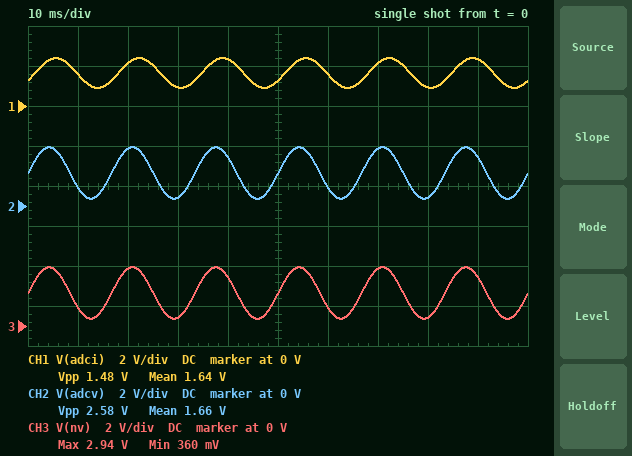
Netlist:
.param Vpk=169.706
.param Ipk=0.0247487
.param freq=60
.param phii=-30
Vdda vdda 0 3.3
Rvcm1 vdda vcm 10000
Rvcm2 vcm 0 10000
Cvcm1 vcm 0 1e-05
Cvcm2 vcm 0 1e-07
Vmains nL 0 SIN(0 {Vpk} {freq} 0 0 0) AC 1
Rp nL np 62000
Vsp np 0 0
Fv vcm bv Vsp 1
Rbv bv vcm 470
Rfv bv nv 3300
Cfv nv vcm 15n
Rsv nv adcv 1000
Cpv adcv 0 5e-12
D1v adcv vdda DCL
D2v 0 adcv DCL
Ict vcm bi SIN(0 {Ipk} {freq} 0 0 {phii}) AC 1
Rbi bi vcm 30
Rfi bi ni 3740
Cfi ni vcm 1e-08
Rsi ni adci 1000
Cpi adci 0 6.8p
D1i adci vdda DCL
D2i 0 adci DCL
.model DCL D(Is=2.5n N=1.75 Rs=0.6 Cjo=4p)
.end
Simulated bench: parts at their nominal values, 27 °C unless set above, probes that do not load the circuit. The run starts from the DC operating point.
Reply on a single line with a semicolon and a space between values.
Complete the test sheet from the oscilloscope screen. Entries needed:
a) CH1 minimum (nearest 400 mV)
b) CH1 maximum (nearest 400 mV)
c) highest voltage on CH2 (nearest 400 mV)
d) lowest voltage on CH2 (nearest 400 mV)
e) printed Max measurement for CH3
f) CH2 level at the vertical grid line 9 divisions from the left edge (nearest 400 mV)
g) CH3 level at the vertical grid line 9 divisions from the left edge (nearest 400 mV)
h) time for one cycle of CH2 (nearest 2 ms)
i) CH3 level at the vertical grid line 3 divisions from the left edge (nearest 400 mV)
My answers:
800 mV; 2.4 V; 2.8 V; 400 mV; 2.94 V; 2.4 V; 2.4 V; 16 ms; 400 mV
